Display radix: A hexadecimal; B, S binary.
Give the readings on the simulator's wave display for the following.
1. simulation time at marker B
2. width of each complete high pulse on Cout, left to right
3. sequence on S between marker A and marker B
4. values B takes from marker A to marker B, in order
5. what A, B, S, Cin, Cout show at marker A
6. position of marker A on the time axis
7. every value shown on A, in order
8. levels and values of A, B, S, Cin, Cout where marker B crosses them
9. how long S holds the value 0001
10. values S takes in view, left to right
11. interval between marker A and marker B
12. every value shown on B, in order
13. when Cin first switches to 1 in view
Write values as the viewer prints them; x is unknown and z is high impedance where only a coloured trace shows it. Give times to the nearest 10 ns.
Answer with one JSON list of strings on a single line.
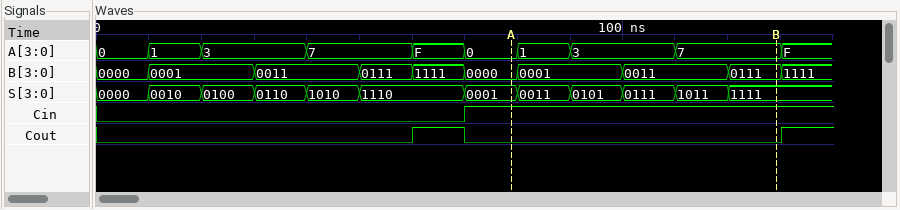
["130 ns", "10 ns", "0001, 0011, 0101, 0111, 1011, 1111", "0000, 0001, 0011, 0111", "A=0, B=0000, S=0001, Cin=1, Cout=0", "80 ns", "0, 1, 3, 7, F, 0, 1, 3, 7, F", "A=7, B=0111, S=1111, Cin=1, Cout=0", "10 ns", "0000, 0010, 0100, 0110, 1010, 1110, 0001, 0011, 0101, 0111, 1011, 1111", "50 ns", "0000, 0001, 0011, 0111, 1111, 0000, 0001, 0011, 0111, 1111", "70 ns"]
